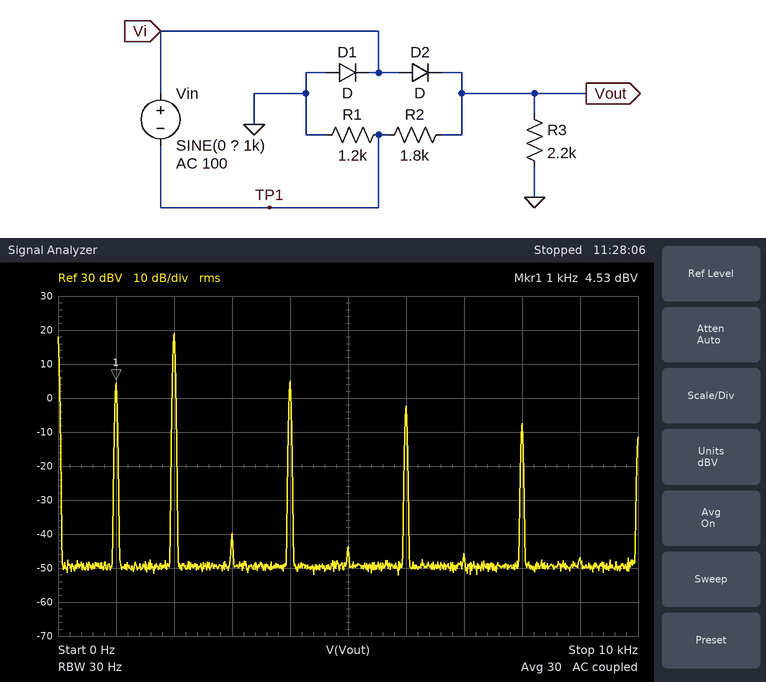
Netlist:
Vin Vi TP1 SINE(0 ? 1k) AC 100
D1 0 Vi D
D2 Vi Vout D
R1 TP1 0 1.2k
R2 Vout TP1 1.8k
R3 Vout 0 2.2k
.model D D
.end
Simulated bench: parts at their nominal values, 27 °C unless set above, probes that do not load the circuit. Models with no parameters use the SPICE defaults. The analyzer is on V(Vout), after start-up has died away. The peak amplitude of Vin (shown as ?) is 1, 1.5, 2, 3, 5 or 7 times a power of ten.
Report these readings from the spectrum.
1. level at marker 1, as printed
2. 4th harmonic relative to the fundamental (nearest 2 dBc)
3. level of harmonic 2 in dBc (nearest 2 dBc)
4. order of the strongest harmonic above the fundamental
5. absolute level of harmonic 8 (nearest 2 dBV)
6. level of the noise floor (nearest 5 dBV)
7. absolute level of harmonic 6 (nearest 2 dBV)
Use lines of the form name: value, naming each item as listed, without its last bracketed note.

level at marker 1, as printed: 4.53 dBV
4th harmonic relative to the fundamental: 0 dBc
level of harmonic 2 in dBc: 14 dBc
order of the strongest harmonic above the fundamental: 2
absolute level of harmonic 8: -8 dBV
level of the noise floor: -50 dBV
absolute level of harmonic 6: -2 dBV
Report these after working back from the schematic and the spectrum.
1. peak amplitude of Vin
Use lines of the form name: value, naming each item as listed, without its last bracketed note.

peak amplitude of Vin: 50 V
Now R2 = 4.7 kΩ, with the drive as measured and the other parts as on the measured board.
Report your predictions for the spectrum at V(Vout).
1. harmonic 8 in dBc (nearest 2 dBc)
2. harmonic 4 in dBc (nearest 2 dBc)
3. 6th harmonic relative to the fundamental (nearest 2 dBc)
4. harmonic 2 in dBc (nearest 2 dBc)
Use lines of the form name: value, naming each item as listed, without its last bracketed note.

harmonic 8 in dBc: -24 dBc
harmonic 4 in dBc: -12 dBc
6th harmonic relative to the fundamental: -20 dBc
harmonic 2 in dBc: 2 dBc
